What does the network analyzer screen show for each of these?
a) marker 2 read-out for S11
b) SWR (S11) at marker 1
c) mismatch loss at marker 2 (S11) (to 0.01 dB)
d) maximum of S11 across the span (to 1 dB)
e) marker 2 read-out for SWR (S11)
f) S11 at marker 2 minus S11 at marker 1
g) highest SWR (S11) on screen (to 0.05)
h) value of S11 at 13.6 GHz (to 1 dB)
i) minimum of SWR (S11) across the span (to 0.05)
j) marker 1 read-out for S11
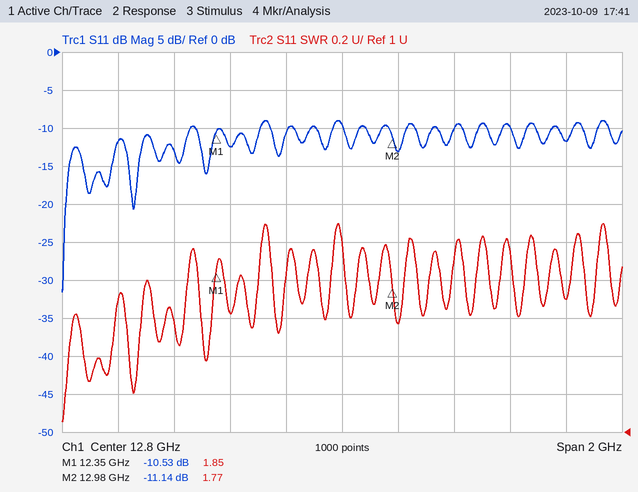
-11.14 dB
1.85
0.35 dB
-9 dB
1.77
-0.61 dB
2.10
-12 dB
1.05
-10.53 dB
